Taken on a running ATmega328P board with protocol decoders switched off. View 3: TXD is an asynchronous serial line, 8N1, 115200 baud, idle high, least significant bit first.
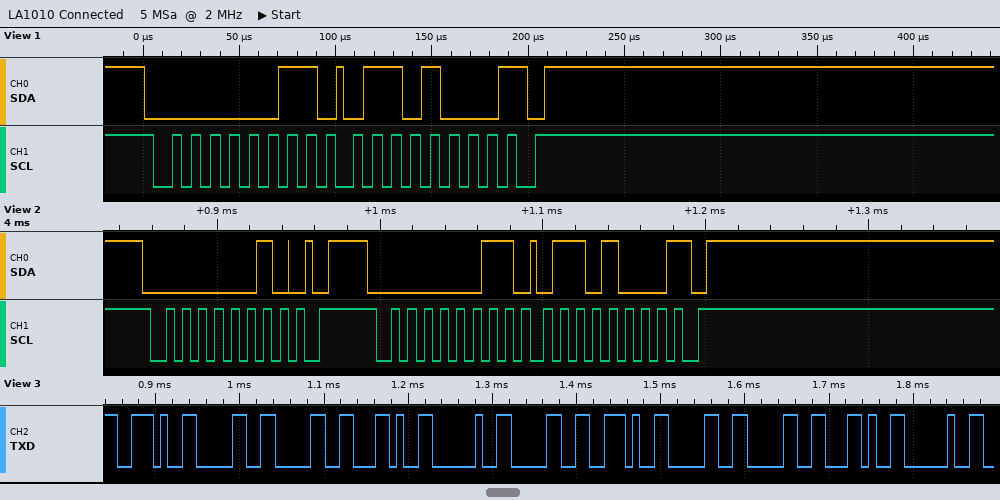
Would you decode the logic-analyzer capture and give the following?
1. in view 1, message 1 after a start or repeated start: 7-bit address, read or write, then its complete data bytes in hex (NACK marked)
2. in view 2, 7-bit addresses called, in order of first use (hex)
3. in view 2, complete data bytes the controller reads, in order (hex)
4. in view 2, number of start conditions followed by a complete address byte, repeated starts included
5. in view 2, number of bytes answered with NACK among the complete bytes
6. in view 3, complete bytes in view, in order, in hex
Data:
0x01 read: 68 NACK
0x01
68
2
1
0x2E 0x30 0x30 0x2C 0x20 0x30 0x2E 0x30 0x30 0x2C 0x20
